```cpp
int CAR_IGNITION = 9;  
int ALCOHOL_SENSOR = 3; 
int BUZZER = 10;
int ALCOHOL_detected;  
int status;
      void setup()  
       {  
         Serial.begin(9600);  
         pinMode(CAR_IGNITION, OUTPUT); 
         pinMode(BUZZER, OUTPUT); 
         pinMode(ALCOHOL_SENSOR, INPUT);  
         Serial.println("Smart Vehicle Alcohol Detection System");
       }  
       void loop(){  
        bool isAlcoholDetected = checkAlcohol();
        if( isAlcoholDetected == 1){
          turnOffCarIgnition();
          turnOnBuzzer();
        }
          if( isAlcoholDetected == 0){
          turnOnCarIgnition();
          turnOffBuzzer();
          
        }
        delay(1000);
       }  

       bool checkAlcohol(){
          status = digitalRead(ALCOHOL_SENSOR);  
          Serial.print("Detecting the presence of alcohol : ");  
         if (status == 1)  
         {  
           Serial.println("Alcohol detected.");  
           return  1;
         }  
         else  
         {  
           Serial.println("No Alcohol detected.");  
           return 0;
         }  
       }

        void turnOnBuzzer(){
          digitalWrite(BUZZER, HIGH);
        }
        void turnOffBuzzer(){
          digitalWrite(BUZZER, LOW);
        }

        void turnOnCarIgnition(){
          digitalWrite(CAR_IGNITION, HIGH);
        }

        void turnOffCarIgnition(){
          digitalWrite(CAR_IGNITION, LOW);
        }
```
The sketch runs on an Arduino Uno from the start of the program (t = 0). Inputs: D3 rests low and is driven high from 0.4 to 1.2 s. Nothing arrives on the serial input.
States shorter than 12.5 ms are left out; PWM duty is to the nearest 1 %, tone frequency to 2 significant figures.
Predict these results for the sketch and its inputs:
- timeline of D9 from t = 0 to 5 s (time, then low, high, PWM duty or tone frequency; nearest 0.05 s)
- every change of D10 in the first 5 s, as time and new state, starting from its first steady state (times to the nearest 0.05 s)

0 s low; 0.05 s high; 1.05 s low; 2.05 s high
0 s low; 1.05 s high; 2.05 s low
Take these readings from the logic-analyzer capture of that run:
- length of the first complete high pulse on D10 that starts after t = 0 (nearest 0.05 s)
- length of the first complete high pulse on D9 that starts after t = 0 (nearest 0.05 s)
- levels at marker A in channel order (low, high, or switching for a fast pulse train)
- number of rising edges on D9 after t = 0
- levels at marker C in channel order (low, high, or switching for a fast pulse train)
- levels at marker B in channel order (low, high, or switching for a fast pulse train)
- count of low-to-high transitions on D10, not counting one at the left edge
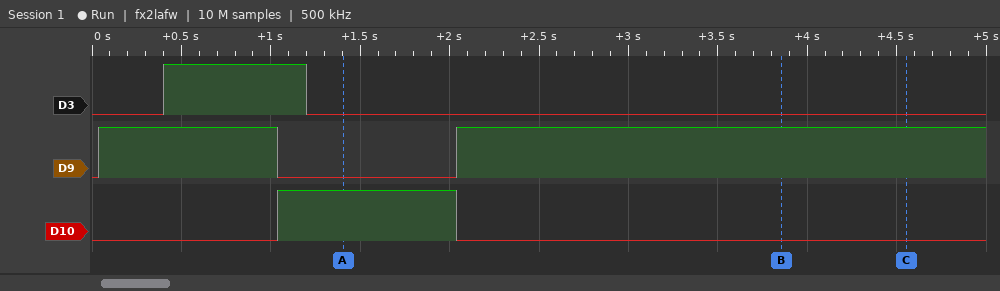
1.00 s
1.00 s
D3 low, D9 low, D10 high
2
D3 low, D9 high, D10 low
D3 low, D9 high, D10 low
1
